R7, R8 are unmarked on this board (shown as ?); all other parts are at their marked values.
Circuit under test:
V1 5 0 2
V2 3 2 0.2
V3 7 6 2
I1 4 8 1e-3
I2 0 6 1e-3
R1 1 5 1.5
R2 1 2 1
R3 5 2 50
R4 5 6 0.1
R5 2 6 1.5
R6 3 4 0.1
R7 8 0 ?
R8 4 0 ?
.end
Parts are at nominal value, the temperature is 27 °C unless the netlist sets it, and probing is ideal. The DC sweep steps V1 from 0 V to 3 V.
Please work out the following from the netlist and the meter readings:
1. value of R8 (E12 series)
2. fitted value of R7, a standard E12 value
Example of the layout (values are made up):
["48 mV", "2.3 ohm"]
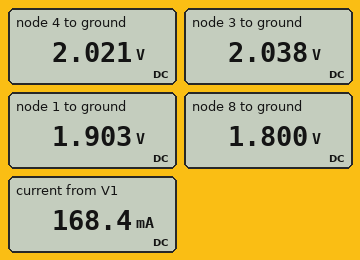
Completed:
["12 Ω", "1.8 kΩ"]
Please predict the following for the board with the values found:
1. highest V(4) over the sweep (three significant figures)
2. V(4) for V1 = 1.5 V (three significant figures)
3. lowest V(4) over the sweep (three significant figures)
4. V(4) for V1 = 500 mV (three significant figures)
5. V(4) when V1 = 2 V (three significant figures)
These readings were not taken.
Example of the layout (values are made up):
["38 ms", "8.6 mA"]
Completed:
["2.94 V", "1.56 V", "183 mV", "642 mV", "2.02 V"]
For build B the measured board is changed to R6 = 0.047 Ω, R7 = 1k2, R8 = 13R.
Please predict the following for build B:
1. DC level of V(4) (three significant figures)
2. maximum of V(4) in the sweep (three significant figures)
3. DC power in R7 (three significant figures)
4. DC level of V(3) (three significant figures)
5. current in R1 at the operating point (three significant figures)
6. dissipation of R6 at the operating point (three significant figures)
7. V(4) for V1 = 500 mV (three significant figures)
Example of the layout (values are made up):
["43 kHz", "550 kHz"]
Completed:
["2.04 V", "2.97 V", "1.20 mW", "2.05 V", "60.5 mA", "1.17 mW", "649 mV"]
